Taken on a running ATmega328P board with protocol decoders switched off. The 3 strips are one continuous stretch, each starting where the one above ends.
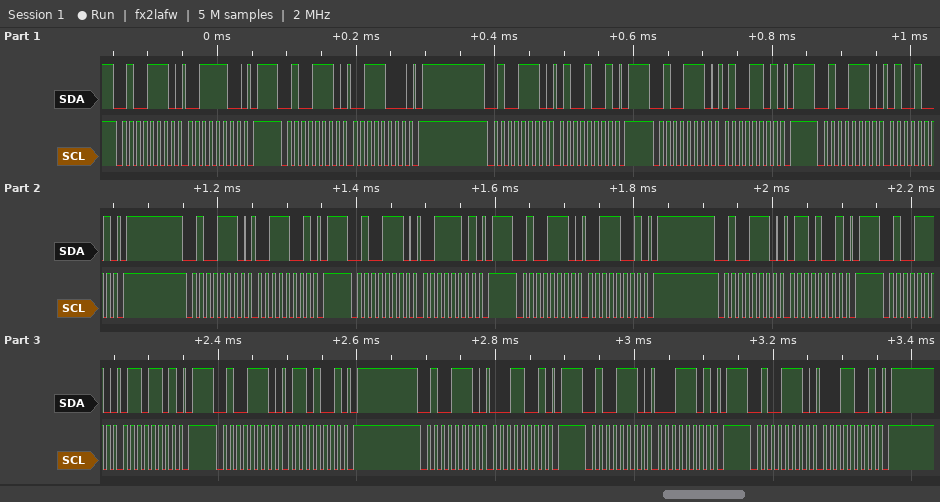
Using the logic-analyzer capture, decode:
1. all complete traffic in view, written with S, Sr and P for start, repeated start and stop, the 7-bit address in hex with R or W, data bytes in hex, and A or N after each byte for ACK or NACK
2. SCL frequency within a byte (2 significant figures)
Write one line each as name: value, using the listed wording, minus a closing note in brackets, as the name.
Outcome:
all complete traffic in view, written with S, Sr and P for start, repeated start and stop, the 7-bit address in hex with R or W, data bytes in hex, and A or N after each byte for ACK or NACK: S 27W A 3C A P S 27W A 38 A P S 27W A 49 A P S 27W A 4D A P S 27W A 49 A P S 27W A 39 A P S 27W A 3D A P S 27W A 39 A P S 27W A 69 A P S 27W A 6D A P S 27W A 69 A P S 27W A 19 A P S 27W A 1D A P S 27W A 19 A P
SCL frequency within a byte: 100 kHz
